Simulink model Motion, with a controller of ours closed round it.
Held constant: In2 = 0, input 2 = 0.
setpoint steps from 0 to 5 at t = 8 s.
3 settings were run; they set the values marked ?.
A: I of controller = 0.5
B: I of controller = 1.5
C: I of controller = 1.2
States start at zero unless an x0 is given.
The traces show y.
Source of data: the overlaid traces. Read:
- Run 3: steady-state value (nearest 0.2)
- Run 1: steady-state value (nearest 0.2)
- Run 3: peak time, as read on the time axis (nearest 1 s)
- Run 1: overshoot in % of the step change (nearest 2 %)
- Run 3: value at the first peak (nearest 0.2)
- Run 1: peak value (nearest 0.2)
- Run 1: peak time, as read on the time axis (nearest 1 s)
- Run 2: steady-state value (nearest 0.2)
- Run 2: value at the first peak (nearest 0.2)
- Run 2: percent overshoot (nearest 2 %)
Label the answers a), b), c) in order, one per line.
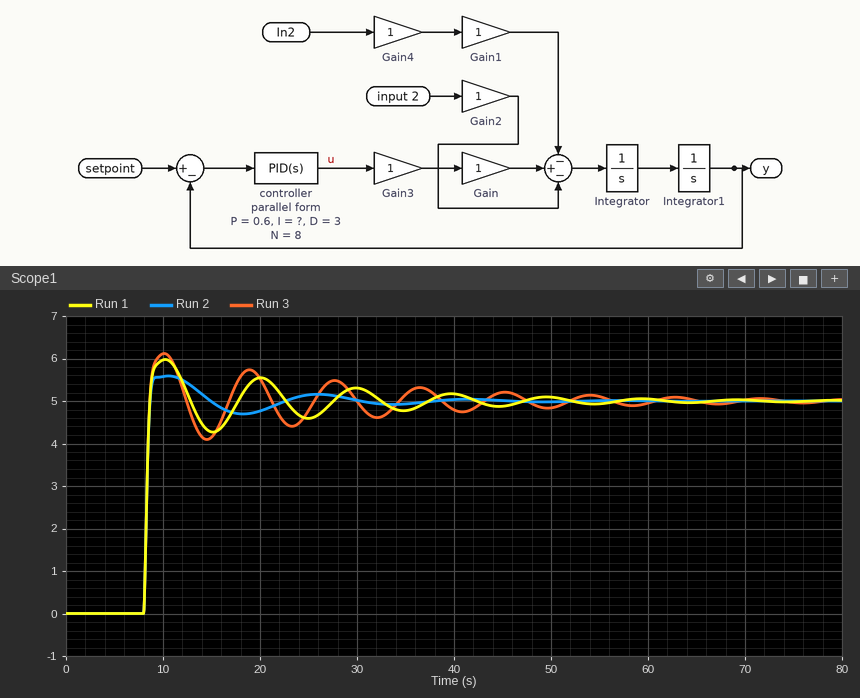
a) 5.0
b) 5.0
c) 10 s
d) 20 %
e) 6.2
f) 6.0
g) 10 s
h) 5.0
i) 5.6
j) 12 %
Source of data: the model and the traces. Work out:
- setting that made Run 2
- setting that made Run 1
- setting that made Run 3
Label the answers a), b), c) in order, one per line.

a) A
b) C
c) B
